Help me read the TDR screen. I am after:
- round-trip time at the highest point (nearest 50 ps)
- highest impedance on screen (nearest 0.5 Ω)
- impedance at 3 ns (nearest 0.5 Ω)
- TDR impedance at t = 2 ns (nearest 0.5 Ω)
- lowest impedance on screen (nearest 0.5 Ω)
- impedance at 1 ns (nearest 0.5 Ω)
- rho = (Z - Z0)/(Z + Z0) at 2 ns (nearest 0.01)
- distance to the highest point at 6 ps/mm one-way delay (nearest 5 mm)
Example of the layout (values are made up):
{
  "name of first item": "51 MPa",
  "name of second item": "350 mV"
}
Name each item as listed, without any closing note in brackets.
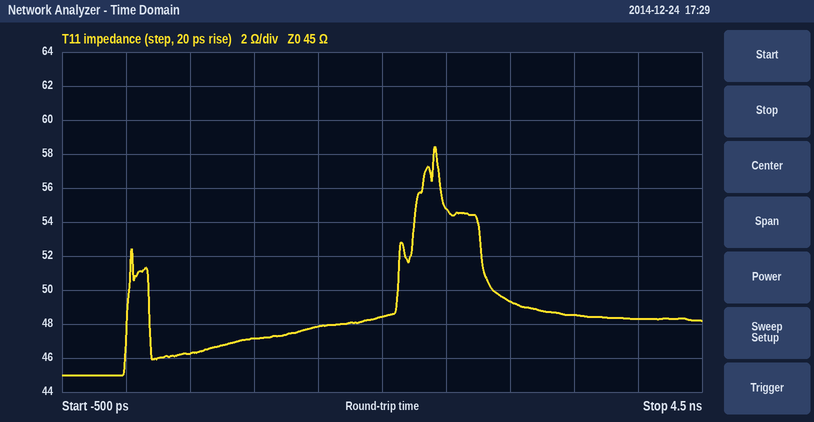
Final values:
{
  "round-trip time at the highest point": "2.40 ns",
  "highest impedance on screen": "58.5 Ω",
  "impedance at 3 ns": "49.5 Ω",
  "TDR impedance at t = 2 ns": "48.5 Ω",
  "lowest impedance on screen": "45.0 Ω",
  "impedance at 1 ns": "47.0 Ω",
  "rho = (Z - Z0)/(Z + Z0) at 2 ns": "+0.04",
  "distance to the highest point at 6 ps/mm one-way delay": "200 mm"
}
